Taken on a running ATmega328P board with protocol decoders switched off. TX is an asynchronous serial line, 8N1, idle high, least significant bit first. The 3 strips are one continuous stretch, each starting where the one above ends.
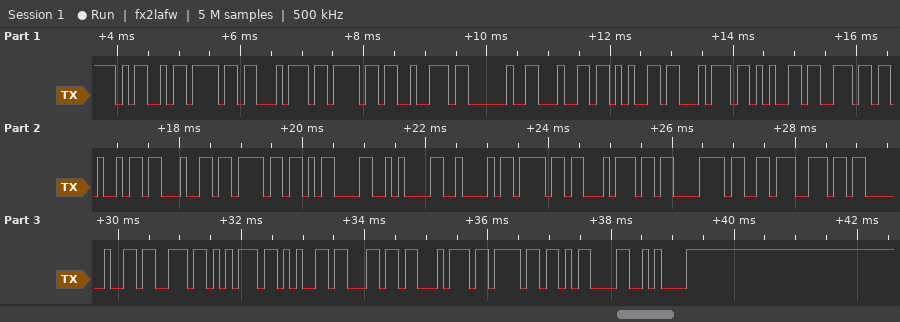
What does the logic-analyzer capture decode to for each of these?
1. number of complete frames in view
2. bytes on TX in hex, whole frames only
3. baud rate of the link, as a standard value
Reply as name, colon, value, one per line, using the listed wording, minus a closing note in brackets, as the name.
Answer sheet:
number of complete frames in view: 31
bytes on TX in hex, whole frames only: 4D 6F 74 6F 72 20 64 65 74 65 6E 69 64 6F 0D 0A 42 6F 74 C3 B3 6E 20 73 75 65 6C 74 6F 0D 0A
baud rate of the link, as a standard value: 9600 baud
